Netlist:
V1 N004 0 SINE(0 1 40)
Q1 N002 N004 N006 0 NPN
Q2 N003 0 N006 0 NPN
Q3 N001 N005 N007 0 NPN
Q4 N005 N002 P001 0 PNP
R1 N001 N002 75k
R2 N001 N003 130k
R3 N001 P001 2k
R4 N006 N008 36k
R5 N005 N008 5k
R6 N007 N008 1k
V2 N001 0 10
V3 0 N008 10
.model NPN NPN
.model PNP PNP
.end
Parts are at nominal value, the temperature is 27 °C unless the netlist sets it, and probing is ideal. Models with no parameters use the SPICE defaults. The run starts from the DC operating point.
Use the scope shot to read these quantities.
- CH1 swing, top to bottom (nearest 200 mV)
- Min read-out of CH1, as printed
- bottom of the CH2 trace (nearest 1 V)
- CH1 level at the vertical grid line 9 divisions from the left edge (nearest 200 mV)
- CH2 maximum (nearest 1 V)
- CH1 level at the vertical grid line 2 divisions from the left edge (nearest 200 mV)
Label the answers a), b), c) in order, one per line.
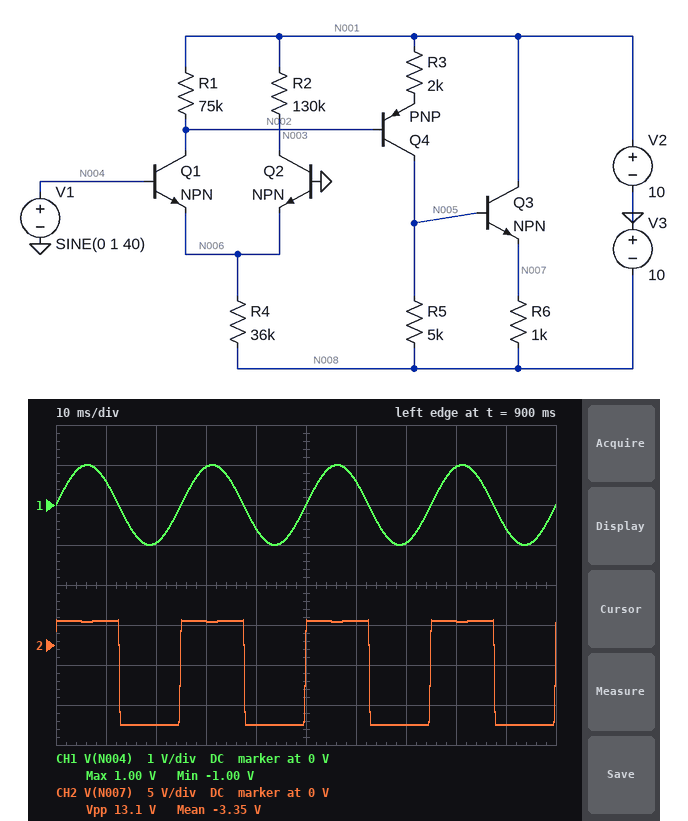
a) 2.0 V
b) -1.00 V
c) -10 V
d) -600 mV
e) 3 V
f) -1.0 V
